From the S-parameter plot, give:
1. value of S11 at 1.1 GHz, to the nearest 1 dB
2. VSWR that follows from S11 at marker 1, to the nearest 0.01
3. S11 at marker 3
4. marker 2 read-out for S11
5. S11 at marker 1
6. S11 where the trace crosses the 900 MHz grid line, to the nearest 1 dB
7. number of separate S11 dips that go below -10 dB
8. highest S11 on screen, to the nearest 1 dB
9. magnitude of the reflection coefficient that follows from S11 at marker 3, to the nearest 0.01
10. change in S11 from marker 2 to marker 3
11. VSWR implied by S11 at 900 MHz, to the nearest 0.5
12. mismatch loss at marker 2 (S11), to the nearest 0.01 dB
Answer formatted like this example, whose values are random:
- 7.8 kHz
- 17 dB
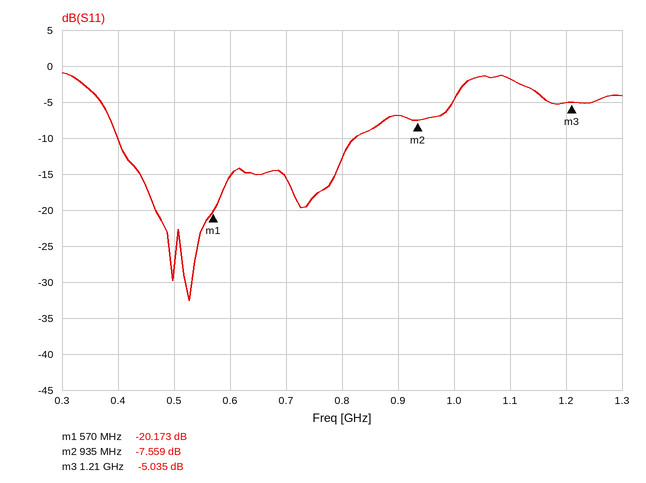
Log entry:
- -2 dB
- 1.22
- -5.035 dB
- -7.559 dB
- -20.173 dB
- -7 dB
- 3
- -1 dB
- 0.56
- 2.524 dB
- 2.5
- 0.84 dB
